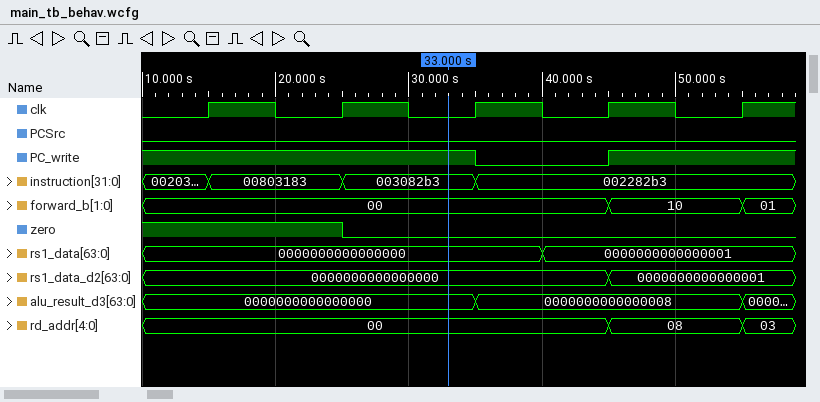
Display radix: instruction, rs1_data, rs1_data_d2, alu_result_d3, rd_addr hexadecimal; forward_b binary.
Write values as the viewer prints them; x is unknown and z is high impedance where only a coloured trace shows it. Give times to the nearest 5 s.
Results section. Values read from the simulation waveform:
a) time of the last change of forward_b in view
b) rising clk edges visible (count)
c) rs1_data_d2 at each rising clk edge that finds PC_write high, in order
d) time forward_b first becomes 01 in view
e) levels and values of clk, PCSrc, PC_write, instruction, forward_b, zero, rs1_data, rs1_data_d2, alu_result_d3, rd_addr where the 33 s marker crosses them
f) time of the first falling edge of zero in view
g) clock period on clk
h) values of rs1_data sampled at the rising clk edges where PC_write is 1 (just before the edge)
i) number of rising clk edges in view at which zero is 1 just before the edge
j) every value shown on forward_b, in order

55 s
5
0000000000000000, 0000000000000000, 0000000000000000, 0000000000000001
55 s
clk=0, PCSrc=0, PC_write=1, instruction=003082b3, forward_b=00, zero=0, rs1_data=0000000000000000, rs1_data_d2=0000000000000000, alu_result_d3=0000000000000000, rd_addr=00
25 s
10 s
0000000000000000, 0000000000000000, 0000000000000000, 0000000000000001
2
00, 10, 01
